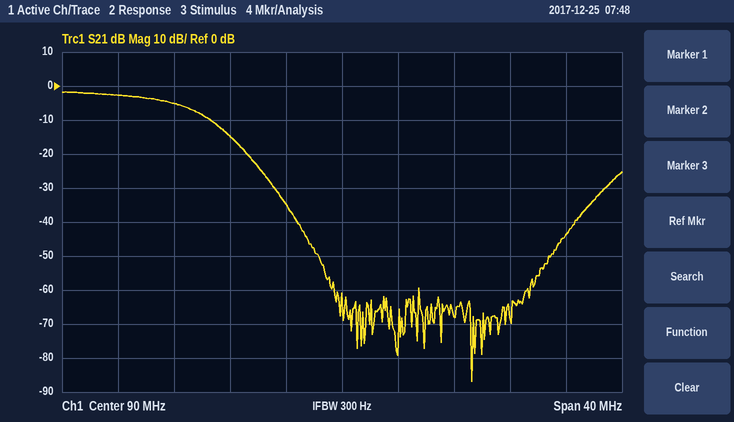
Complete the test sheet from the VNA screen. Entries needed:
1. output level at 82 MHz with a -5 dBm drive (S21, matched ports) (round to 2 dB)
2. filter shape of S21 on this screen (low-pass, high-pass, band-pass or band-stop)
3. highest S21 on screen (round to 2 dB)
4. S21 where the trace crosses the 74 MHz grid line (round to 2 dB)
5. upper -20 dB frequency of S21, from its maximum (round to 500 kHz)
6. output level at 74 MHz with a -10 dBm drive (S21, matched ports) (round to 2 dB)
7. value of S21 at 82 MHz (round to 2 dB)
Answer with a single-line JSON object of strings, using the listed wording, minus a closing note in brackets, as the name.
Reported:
{"output level at 82 MHz with a -5 dBm drive (S21, matched ports)": "-20 dBm", "filter shape of S21 on this screen": "low-pass", "highest S21 on screen": "-2 dB", "S21 where the trace crosses the 74 MHz grid line": "-2 dB", "upper -20 dB frequency of S21, from its maximum": "83.5 MHz", "output level at 74 MHz with a -10 dBm drive (S21, matched ports)": "-12 dBm", "value of S21 at 82 MHz": "-14 dB"}
